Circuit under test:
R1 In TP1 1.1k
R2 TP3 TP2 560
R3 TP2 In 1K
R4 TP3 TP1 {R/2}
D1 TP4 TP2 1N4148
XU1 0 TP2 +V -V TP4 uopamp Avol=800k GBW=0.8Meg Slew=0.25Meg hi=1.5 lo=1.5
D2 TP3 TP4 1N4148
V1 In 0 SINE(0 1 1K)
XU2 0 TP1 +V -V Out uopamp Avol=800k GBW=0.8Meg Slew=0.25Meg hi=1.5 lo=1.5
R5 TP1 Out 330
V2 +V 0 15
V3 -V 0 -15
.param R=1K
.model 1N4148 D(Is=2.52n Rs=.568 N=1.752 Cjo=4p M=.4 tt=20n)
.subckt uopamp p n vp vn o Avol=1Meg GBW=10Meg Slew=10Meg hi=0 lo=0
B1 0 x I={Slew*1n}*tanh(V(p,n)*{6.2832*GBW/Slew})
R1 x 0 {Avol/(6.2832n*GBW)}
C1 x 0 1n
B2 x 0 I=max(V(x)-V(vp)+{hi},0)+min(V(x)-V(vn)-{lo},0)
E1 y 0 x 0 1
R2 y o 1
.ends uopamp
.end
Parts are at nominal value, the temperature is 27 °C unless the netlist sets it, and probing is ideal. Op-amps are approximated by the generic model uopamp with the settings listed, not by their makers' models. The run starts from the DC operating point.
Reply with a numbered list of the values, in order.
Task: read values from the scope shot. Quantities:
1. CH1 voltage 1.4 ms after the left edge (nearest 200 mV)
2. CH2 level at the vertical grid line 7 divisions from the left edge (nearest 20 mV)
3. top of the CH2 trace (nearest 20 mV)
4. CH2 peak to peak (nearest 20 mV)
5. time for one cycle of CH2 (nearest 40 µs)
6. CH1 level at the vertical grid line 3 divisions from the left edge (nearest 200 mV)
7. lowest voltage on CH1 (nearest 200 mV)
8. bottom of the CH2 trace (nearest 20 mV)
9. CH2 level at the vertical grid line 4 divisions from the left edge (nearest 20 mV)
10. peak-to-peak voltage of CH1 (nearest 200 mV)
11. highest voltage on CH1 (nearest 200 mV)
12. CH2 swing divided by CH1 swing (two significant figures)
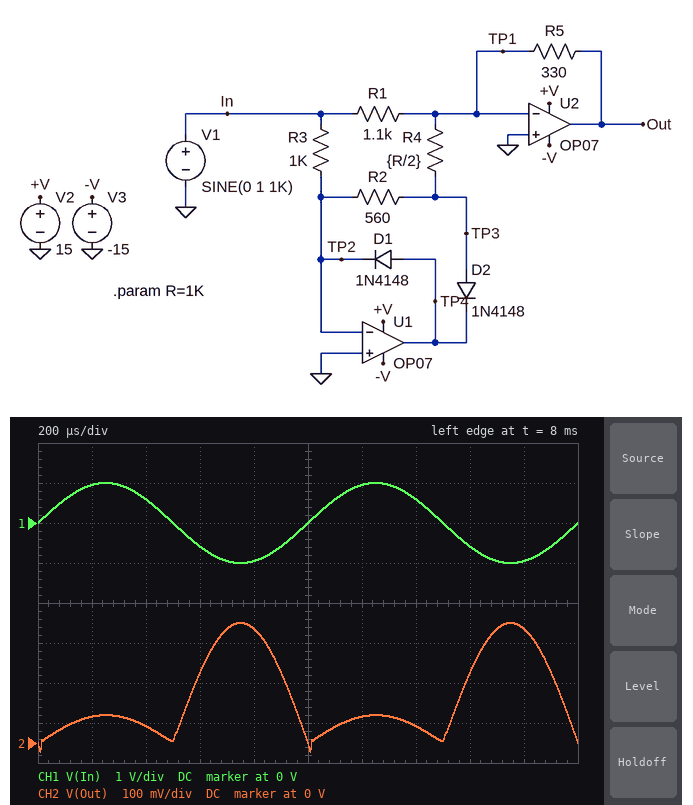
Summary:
1. 600 mV
2. 40 mV
3. 300 mV
4. 320 mV
5. 1.00 ms
6. -600 mV
7. -1.0 V
8. -20 mV
9. 280 mV
10. 2.0 V
11. 1.0 V
12. 0.16
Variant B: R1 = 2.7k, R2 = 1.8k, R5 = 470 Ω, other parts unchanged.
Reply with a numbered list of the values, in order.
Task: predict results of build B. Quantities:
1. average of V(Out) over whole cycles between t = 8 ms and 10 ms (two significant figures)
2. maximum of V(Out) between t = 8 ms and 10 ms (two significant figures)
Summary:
1. 540 mV
2. 1.5 V
